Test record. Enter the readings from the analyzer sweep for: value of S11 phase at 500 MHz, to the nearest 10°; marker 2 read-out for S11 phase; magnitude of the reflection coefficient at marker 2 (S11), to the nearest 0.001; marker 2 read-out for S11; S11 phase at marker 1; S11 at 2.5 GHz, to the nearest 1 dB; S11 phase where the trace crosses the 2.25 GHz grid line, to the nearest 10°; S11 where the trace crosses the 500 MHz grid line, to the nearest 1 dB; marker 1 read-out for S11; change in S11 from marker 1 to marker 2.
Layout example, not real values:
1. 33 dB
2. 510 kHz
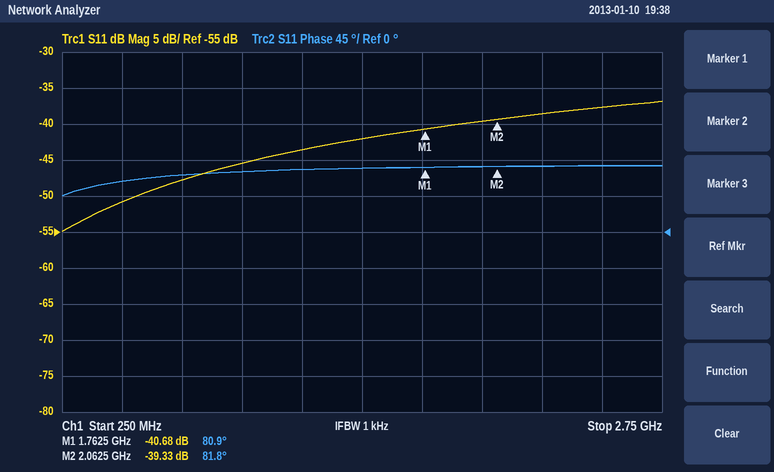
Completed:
1. 60°
2. 81.8°
3. 0.011
4. -39.33 dB
5. 80.9°
6. -38 dB
7. 80°
8. -51 dB
9. -40.68 dB
10. 1.35 dB
